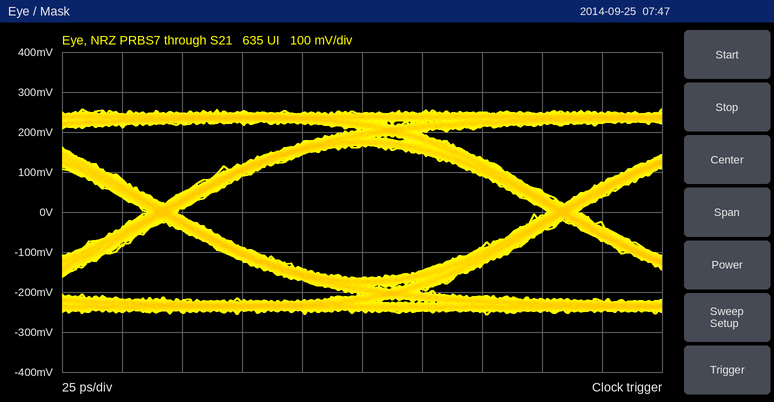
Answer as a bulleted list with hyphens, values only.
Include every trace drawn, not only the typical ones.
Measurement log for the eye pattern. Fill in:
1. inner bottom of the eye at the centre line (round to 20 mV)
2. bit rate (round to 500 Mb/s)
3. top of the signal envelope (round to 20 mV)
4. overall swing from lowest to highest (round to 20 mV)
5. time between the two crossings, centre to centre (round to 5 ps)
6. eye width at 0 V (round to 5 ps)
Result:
- -160 mV
- 6.0 Gb/s
- 260 mV
- 520 mV
- 165 ps
- 155 ps
